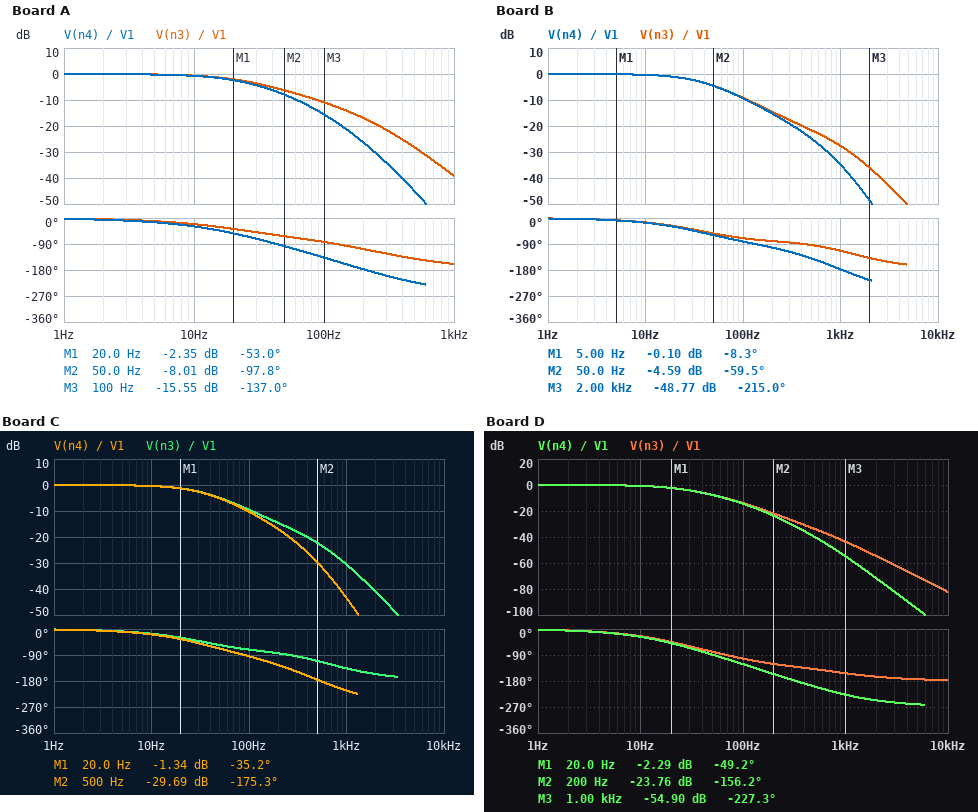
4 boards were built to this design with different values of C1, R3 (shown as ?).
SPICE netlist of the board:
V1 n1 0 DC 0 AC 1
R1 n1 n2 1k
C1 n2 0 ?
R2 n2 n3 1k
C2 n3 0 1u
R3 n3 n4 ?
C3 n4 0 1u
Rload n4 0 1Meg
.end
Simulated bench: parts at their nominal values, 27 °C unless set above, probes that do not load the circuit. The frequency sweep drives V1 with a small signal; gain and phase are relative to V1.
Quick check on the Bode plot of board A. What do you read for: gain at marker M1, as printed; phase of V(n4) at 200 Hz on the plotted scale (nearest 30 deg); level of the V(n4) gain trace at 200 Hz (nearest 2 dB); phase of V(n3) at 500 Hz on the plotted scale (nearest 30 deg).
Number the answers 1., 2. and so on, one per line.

1. -2.35 dB
2. -180 deg
3. -26 dB
4. -150 deg
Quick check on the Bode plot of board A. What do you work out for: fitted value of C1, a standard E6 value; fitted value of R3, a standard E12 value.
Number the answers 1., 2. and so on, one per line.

1. 2.2 µF
2. 2.2 kΩ
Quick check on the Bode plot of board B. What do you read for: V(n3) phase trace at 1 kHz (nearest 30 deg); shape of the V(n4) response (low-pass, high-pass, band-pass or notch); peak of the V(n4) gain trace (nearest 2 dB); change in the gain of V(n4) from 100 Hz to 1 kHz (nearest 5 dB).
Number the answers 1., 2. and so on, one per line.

1. -120 deg
2. low-pass
3. 0 dB
4. -25 dB
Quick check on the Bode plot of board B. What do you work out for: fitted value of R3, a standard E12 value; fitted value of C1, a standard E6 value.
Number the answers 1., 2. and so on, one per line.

1. 330 Ω
2. 330 nF
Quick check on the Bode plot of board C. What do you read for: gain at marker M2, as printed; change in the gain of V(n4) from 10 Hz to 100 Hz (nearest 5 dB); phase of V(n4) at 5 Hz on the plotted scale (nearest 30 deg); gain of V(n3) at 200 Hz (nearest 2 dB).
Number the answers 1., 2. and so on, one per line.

1. -29.69 dB
2. -10 dB
3. 0 deg
4. -14 dB
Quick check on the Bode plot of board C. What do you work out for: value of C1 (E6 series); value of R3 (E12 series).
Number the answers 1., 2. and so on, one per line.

1. 680 nF
2. 680 Ω
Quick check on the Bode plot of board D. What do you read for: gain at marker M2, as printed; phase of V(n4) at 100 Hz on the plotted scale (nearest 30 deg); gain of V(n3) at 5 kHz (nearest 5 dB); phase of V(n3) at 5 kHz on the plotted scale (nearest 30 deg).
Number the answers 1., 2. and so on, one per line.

1. -23.76 dB
2. -120 deg
3. -70 dB
4. -180 deg
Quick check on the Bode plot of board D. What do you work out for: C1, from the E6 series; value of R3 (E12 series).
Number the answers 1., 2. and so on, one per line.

1. 3.3 µF
2. 560 Ω
